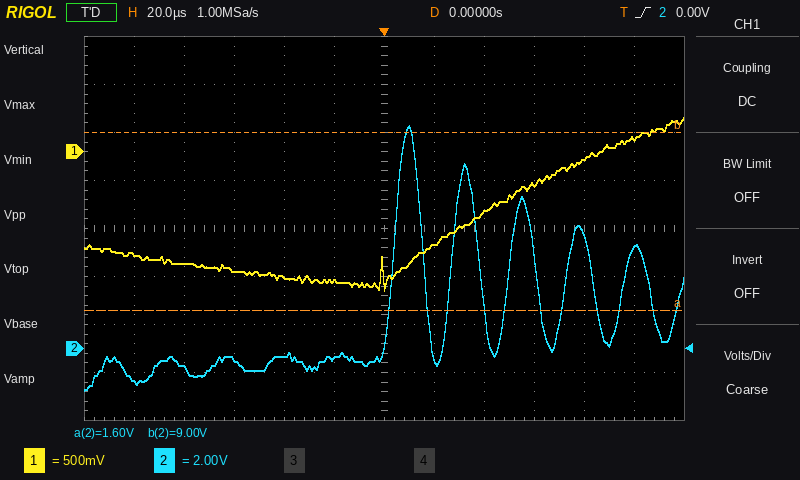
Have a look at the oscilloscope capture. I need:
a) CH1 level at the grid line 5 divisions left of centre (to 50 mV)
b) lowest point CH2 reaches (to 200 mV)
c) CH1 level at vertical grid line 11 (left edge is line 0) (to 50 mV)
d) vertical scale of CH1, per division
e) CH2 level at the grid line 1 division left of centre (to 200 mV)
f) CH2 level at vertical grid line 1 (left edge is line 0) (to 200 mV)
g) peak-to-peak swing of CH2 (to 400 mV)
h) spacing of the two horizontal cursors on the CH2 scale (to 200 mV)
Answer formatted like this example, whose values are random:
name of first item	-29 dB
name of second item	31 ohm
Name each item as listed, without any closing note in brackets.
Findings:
CH1 level at the grid line 5 divisions left of centre	-1.05 V
lowest point CH2 reaches	-1.8 V
CH1 level at vertical grid line 11 (left edge is line 0)	150 mV
vertical scale of CH1, per division	500 mV
CH2 level at the grid line 1 division left of centre	-400 mV
CH2 level at vertical grid line 1 (left edge is line 0)	-1.4 V
peak-to-peak swing of CH2	11.2 V
spacing of the two horizontal cursors on the CH2 scale	7.4 V
